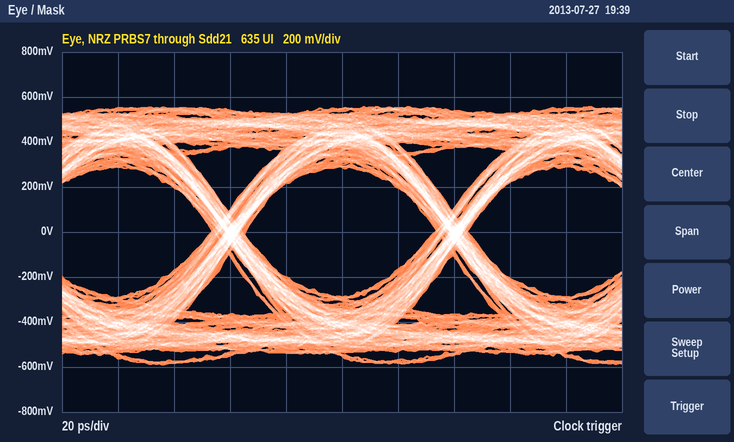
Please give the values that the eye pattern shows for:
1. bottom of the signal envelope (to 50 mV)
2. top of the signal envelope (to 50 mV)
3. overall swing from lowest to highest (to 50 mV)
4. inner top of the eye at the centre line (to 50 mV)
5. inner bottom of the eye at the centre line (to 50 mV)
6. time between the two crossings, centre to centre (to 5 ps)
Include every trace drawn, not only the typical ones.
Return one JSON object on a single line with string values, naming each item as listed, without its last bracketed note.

{"bottom of the signal envelope": "-600 mV", "top of the signal envelope": "550 mV", "overall swing from lowest to highest": "1.15 V", "inner top of the eye at the centre line": "300 mV", "inner bottom of the eye at the centre line": "-300 mV", "time between the two crossings, centre to centre": "80 ps"}
